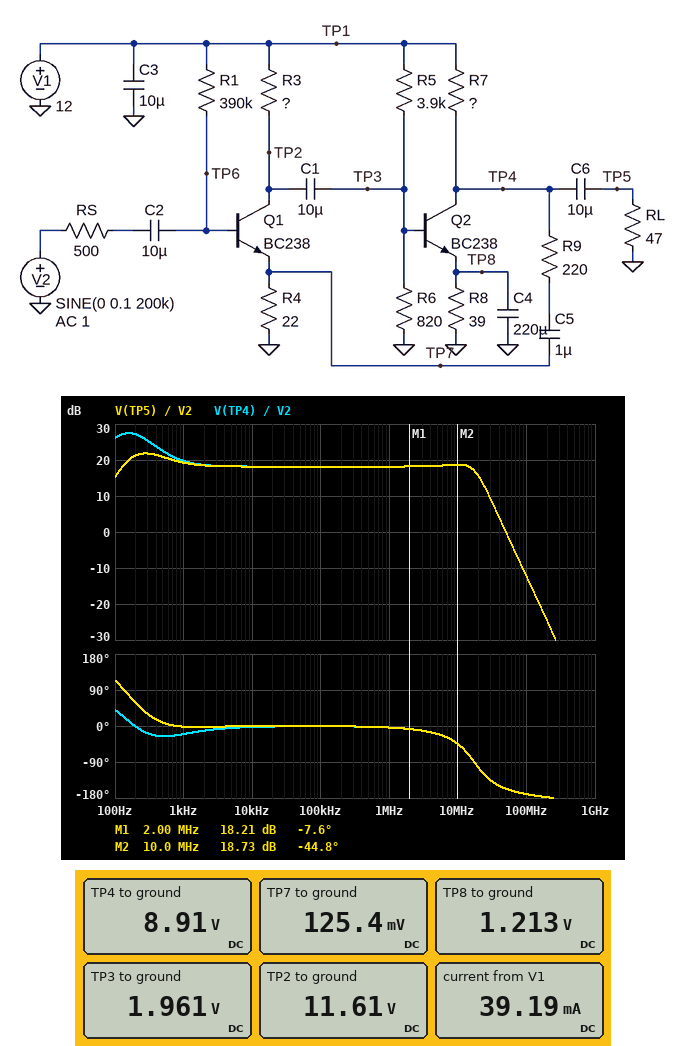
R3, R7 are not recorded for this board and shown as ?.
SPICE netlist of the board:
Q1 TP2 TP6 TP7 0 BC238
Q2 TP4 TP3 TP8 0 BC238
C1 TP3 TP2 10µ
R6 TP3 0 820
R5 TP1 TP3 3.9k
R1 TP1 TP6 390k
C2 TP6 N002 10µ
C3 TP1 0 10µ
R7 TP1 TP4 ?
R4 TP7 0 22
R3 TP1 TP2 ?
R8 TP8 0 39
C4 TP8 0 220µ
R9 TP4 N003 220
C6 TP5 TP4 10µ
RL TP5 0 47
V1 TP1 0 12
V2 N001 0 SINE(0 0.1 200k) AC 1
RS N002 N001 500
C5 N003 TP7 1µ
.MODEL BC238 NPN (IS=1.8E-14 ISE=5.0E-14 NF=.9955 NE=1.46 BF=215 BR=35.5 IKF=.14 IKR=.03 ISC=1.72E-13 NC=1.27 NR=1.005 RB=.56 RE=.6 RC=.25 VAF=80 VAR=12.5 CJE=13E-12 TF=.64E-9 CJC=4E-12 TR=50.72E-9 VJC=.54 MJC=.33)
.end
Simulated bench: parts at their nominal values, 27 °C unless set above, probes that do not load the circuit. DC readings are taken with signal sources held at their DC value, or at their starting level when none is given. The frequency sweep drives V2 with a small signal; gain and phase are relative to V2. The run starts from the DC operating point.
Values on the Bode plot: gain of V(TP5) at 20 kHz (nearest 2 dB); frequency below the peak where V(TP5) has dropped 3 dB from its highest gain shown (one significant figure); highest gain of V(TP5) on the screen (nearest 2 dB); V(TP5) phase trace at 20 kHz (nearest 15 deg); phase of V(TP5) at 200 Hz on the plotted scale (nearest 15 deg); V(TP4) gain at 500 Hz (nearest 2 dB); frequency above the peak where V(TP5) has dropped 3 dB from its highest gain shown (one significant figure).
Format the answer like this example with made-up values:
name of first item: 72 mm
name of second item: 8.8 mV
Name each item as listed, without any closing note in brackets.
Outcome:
gain of V(TP5) at 20 kHz: 18 dB
frequency below the peak where V(TP5) has dropped 3 dB from its highest gain shown: 100 Hz
highest gain of V(TP5) on the screen: 22 dB
V(TP5) phase trace at 20 kHz: 0 deg
phase of V(TP5) at 200 Hz on the plotted scale: 60 deg
V(TP4) gain at 500 Hz: 22 dB
frequency above the peak where V(TP5) has dropped 3 dB from its highest gain shown: 1 kHz
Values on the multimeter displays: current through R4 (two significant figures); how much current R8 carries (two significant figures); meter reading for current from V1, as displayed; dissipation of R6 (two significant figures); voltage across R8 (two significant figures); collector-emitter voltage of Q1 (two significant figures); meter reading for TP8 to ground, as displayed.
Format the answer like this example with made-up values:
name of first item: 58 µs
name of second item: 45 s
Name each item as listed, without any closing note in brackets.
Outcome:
current through R4: 5.7 mA
how much current R8 carries: 31 mA
meter reading for current from V1, as displayed: 39.19 mA
dissipation of R6: 4.7 mW
voltage across R8: 1.2 V
collector-emitter voltage of Q1: 11 V
meter reading for TP8 to ground, as displayed: 1.213 V
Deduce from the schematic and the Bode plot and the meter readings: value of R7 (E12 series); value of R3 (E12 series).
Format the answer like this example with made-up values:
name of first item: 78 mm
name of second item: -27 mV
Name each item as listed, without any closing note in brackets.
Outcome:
value of R7: 100 Ω
value of R3: 68 Ω
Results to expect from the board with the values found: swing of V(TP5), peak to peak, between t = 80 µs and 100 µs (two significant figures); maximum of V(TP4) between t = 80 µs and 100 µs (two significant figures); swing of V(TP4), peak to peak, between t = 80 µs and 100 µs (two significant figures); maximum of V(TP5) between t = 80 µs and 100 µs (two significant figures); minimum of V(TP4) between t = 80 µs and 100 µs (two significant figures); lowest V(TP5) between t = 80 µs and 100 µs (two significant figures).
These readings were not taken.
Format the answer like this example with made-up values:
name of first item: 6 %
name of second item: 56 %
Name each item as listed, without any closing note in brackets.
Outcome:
swing of V(TP5), peak to peak, between t = 80 µs and 100 µs: 1.6 V
maximum of V(TP4) between t = 80 µs and 100 µs: 9.6 V
swing of V(TP4), peak to peak, between t = 80 µs and 100 µs: 1.6 V
maximum of V(TP5) between t = 80 µs and 100 µs: 730 mV
minimum of V(TP4) between t = 80 µs and 100 µs: 8.1 V
lowest V(TP5) between t = 80 µs and 100 µs: -830 mV
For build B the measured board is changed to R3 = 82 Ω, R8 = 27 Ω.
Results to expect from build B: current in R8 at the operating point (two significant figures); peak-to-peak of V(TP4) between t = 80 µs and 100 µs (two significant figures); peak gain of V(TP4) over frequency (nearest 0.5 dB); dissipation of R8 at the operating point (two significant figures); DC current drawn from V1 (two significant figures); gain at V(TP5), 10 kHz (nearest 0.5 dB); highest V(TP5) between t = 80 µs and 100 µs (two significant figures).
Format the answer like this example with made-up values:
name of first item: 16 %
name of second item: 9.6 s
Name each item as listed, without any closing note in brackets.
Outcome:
current in R8 at the operating point: 42 mA
peak-to-peak of V(TP4) between t = 80 µs and 100 µs: 1.7 V
peak gain of V(TP4) over frequency: 28.5 dB
dissipation of R8 at the operating point: 48 mW
DC current drawn from V1: 50 mA
gain at V(TP5), 10 kHz: 18.5 dB
highest V(TP5) between t = 80 µs and 100 µs: 820 mV
